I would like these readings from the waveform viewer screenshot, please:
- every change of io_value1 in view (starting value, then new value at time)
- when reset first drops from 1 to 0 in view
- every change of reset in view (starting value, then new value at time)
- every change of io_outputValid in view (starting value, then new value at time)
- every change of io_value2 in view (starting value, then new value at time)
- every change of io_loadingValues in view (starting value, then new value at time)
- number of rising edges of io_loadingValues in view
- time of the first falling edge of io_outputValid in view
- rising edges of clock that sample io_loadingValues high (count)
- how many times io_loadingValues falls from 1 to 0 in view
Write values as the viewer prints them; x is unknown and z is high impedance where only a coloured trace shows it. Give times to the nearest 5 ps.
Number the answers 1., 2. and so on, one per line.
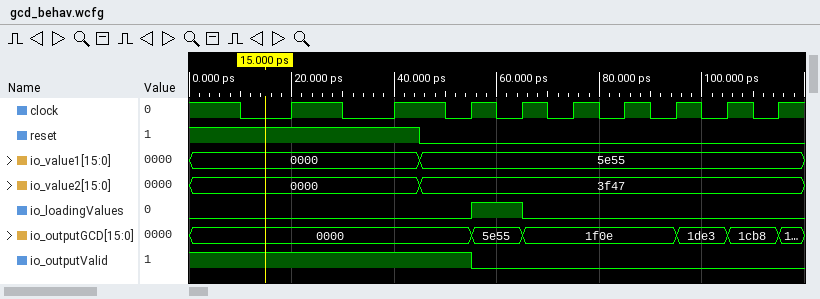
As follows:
1. 0000, 5e55 at 45 ps
2. 45 ps
3. 1, 0 at 45 ps
4. 1, 0 at 55 ps
5. 0000, 3f47 at 45 ps
6. 0, 1 at 55 ps, 0 at 65 ps
7. 1
8. 55 ps
9. 1
10. 1
